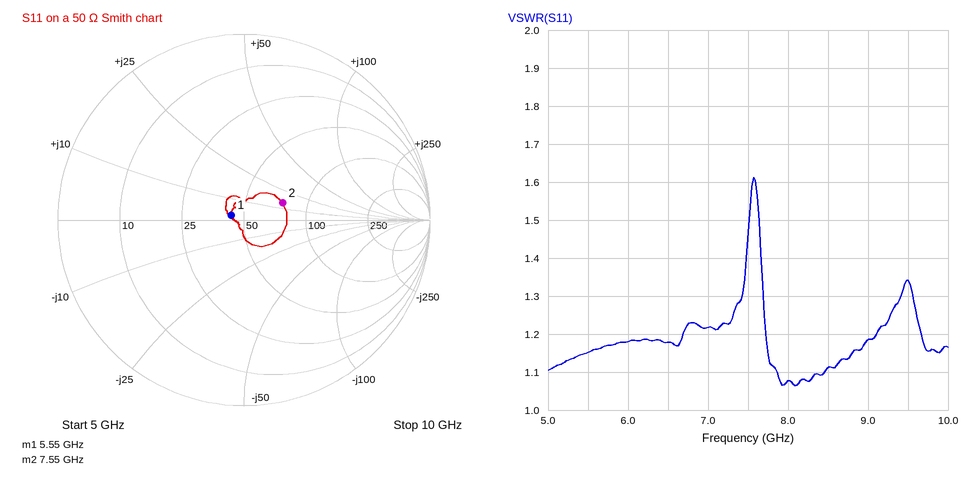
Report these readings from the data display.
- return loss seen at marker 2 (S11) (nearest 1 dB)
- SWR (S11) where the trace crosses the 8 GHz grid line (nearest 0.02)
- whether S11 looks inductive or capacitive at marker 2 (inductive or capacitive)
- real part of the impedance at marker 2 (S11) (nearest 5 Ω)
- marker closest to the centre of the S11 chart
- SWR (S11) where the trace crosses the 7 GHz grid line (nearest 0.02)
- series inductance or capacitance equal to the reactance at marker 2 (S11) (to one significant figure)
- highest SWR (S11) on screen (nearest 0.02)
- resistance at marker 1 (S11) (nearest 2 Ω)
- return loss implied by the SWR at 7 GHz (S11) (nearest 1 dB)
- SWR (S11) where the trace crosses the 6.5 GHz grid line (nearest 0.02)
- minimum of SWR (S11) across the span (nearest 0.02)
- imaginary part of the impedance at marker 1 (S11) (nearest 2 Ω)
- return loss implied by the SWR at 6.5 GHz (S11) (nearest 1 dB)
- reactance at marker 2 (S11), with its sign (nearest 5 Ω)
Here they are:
13 dB
1.08
inductive
75 Ω
marker 1
1.22
300 pH
1.62
44 Ω
20 dB
1.18
1.06
+2 Ω
22 dB
+15 Ω
